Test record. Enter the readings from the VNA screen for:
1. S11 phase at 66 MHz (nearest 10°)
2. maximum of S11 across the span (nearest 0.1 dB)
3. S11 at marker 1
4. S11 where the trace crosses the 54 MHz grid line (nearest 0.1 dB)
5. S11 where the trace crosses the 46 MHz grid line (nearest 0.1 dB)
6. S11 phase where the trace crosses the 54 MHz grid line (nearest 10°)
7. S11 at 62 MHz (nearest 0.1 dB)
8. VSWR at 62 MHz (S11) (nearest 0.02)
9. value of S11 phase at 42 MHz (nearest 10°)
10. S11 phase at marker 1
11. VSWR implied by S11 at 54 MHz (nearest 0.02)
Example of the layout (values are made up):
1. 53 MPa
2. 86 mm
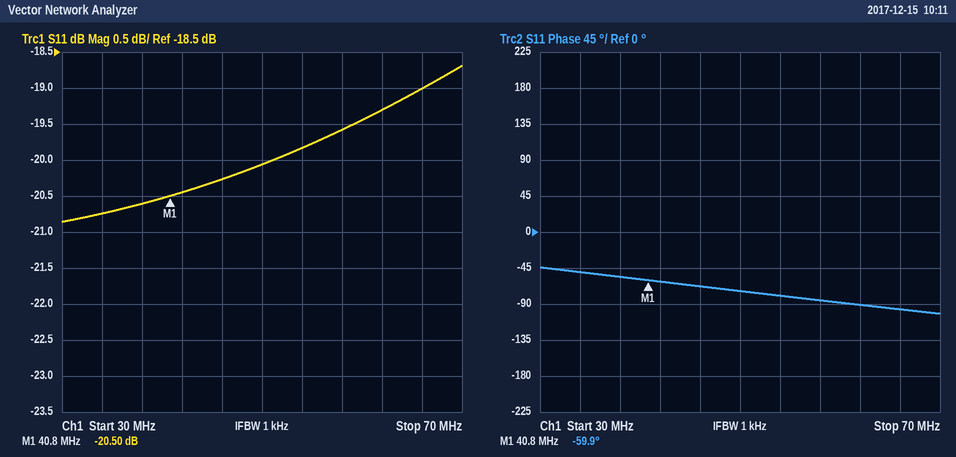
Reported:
1. -100°
2. -18.7 dB
3. -20.50 dB
4. -19.8 dB
5. -20.3 dB
6. -80°
7. -19.3 dB
8. 1.24
9. -60°
10. -59.9°
11. 1.22
